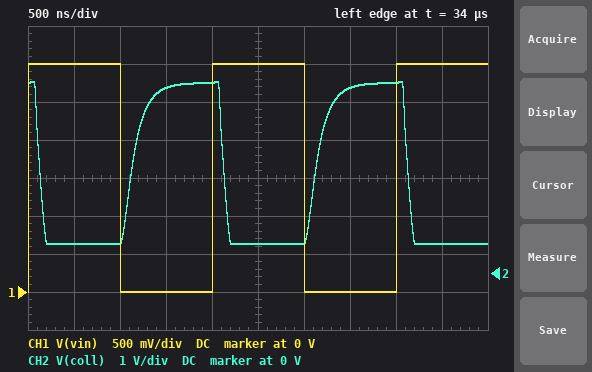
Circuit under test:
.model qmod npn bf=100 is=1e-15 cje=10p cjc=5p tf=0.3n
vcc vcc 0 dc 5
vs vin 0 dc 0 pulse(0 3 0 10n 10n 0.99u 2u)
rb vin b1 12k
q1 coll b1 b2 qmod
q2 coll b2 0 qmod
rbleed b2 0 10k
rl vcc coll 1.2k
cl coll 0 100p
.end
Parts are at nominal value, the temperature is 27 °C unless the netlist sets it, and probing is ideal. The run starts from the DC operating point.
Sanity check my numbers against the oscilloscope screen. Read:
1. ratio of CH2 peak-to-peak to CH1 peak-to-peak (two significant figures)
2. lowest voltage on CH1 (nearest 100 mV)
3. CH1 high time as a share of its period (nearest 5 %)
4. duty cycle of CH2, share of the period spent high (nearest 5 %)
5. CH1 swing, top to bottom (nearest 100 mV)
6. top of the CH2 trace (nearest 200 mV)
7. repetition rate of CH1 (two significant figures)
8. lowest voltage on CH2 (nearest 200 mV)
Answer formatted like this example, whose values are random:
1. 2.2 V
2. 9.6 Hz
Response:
1. 1.4
2. 0 V
3. 50 %
4. 50 %
5. 3.0 V
6. 5.0 V
7. 500 kHz
8. 800 mV
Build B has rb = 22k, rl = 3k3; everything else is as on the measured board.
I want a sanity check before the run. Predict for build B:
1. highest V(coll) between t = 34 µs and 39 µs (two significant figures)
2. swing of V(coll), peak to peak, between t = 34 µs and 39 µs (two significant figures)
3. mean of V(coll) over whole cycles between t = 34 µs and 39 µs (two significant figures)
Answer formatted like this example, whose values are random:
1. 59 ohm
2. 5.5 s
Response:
1. 4.8 V
2. 4.1 V
3. 2.5 V
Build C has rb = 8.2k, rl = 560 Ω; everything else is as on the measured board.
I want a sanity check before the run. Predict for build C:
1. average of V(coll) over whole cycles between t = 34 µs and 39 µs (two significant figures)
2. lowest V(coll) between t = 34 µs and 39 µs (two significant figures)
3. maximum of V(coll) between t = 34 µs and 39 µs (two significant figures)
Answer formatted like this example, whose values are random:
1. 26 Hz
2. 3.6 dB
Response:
1. 2.9 V
2. 770 mV
3. 5.0 V
